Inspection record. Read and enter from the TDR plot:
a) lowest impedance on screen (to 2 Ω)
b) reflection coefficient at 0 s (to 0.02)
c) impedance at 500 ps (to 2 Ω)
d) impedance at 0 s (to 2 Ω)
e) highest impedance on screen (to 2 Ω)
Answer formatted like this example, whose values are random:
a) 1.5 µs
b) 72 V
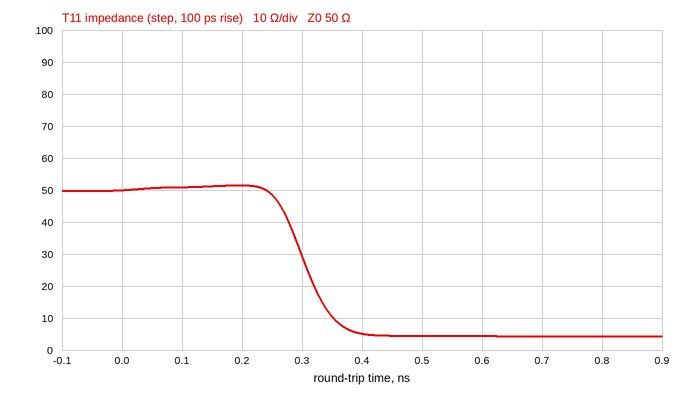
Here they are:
a) 4 Ω
b) 0.00
c) 4 Ω
d) 50 Ω
e) 52 Ω
